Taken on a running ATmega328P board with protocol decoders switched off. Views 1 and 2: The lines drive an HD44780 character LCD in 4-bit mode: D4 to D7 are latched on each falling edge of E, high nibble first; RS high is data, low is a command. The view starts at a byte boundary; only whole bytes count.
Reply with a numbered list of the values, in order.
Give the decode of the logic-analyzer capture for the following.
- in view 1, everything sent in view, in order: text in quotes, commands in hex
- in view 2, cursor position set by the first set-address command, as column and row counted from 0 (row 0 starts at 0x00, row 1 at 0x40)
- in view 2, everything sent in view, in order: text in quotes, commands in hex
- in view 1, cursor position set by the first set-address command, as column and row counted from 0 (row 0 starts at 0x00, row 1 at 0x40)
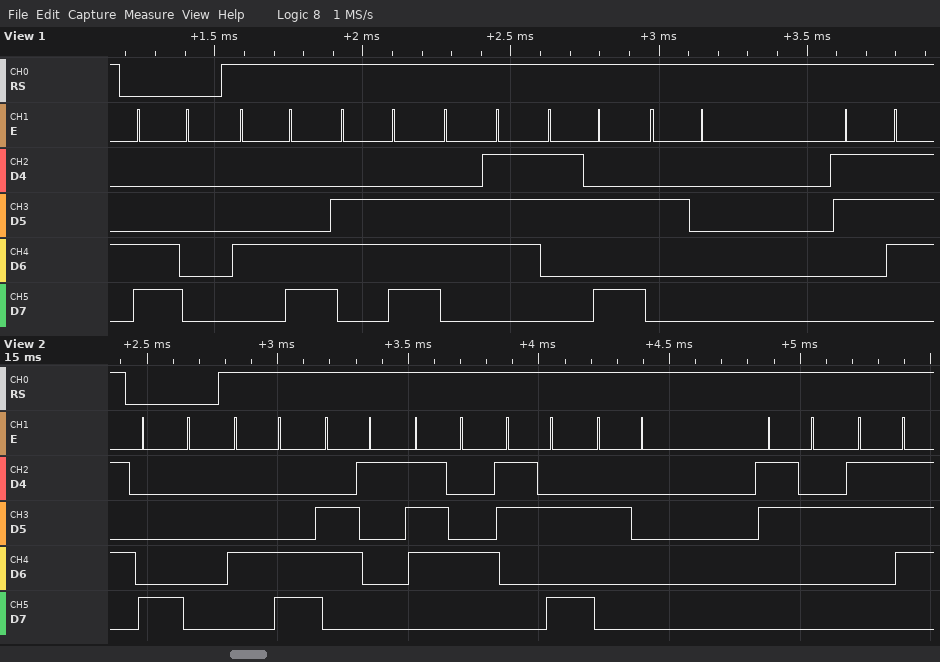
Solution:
1. 0xC0 "Lng: 7"
2. column 0, row 0
3. 0x80 "Lat: 27"
4. column 0, row 1
